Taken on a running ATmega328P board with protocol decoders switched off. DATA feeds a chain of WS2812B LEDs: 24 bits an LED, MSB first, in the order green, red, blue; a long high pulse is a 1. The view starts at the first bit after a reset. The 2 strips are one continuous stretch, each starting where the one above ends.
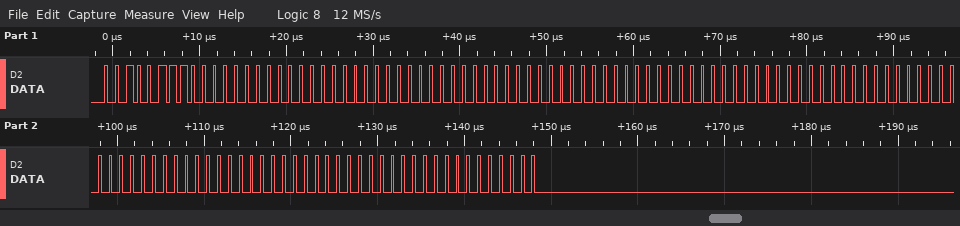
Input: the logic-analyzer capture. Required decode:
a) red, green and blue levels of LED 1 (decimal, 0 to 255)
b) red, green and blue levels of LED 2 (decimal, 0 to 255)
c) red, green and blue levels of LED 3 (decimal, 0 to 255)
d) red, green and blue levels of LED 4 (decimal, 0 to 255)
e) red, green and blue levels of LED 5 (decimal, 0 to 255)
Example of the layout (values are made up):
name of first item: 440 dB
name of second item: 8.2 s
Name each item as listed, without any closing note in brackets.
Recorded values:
red, green and blue levels of LED 1: 0, 39, 0
red, green and blue levels of LED 2: 0, 0, 0
red, green and blue levels of LED 3: 0, 0, 0
red, green and blue levels of LED 4: 0, 0, 0
red, green and blue levels of LED 5: 0, 0, 0
